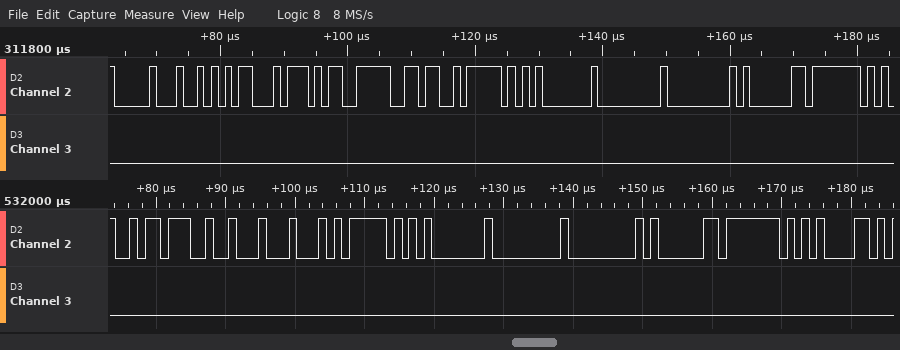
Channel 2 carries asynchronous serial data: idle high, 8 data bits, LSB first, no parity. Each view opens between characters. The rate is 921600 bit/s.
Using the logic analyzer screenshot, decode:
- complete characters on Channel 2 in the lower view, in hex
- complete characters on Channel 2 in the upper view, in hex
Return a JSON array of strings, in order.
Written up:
["DA, 12, 44, 5F, 01, 00, 00, 81, 7F, 85", "10, AA, 74, F3, 36, 5F, 01, 00, 00, 81, 7F"]
